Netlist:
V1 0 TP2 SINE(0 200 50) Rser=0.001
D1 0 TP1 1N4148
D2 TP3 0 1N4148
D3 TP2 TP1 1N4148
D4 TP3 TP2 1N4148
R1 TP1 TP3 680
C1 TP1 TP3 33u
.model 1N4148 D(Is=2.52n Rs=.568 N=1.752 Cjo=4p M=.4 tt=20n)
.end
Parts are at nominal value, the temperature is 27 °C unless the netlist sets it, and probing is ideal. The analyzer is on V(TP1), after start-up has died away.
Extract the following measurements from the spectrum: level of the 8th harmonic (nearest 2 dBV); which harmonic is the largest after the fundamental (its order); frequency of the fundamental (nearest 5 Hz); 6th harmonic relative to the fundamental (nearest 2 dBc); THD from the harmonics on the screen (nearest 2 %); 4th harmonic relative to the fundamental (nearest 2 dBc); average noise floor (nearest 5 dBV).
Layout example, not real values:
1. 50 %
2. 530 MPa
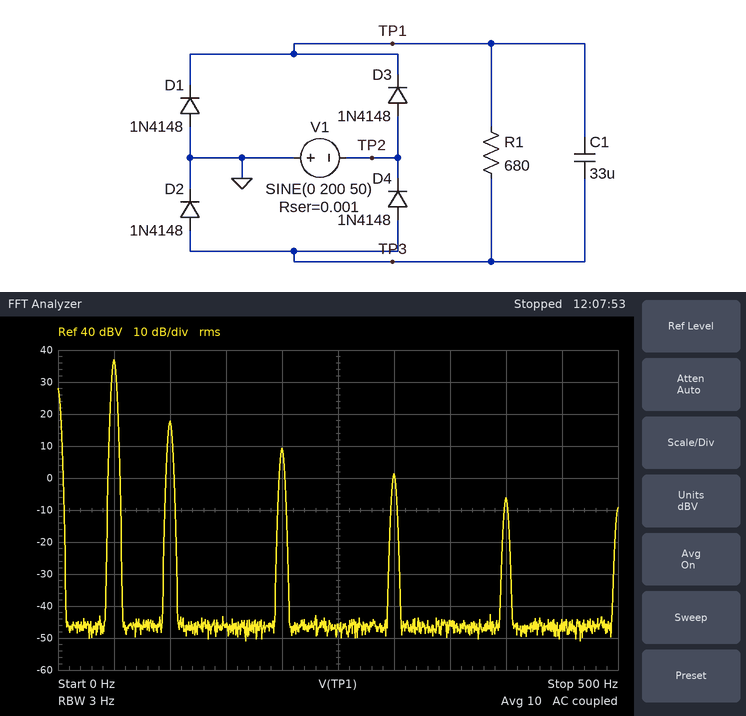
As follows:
1. -6 dBV
2. 2
3. 50 Hz
4. -36 dBc
5. 12 %
6. -28 dBc
7. -45 dBV
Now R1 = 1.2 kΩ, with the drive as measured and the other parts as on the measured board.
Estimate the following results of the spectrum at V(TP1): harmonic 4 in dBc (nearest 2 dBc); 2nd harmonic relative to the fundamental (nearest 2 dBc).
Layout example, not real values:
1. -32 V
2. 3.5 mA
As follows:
1. -30 dBc
2. -24 dBc
